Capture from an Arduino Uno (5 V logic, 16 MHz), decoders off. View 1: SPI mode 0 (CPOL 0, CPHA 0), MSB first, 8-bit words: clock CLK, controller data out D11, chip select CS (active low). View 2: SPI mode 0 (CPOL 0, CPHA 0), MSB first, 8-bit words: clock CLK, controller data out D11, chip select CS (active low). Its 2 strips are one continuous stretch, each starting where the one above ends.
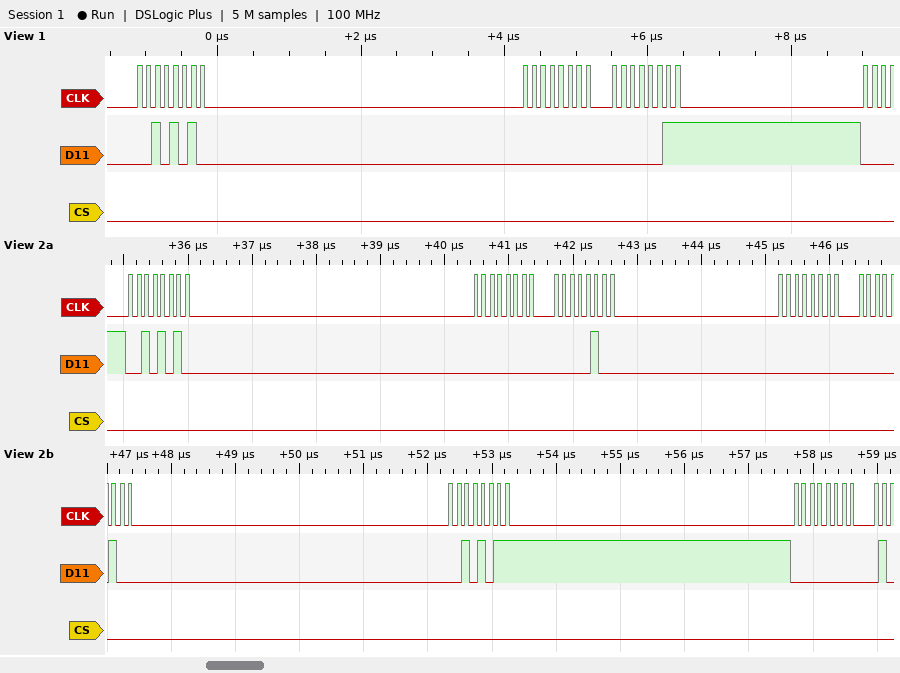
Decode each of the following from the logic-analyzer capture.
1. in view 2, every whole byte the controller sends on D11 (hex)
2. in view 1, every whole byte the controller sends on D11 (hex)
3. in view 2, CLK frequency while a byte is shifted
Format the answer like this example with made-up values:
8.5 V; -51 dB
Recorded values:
0x2A 0x00 0x04 0x00 0x04 0x2B 0x00; 2A 00 03; 8 MHz
